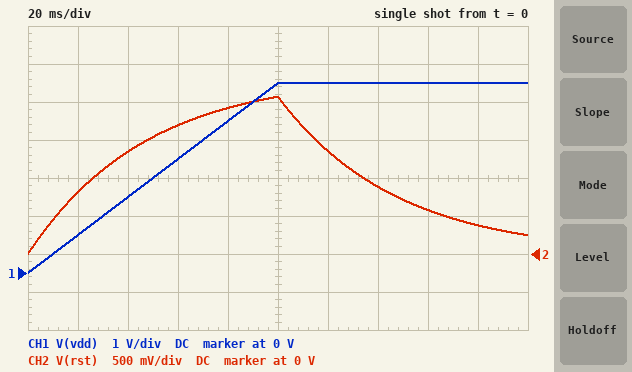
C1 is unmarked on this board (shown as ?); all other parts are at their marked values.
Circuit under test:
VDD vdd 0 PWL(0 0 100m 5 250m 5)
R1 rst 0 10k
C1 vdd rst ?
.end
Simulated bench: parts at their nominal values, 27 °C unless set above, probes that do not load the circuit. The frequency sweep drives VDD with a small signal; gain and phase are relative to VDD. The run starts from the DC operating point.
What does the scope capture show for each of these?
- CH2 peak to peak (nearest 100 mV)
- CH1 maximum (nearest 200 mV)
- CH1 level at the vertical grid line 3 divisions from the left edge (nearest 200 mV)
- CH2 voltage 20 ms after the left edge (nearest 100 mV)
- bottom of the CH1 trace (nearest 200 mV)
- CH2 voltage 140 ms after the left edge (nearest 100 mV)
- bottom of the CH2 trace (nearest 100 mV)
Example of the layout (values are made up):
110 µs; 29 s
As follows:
2.1 V; 5.0 V; 3.0 V; 800 mV; 0 V; 900 mV; 0 V
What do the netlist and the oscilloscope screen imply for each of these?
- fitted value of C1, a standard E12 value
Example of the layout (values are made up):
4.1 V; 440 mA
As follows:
4.7 µF
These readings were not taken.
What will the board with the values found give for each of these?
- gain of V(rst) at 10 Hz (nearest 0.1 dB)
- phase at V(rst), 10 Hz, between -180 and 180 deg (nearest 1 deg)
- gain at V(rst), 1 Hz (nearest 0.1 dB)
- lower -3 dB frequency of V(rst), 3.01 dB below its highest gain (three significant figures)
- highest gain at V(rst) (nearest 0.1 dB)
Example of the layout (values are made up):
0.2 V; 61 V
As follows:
-0.5 dB; 19 deg; -11.0 dB; 3.39 Hz; 0 dB
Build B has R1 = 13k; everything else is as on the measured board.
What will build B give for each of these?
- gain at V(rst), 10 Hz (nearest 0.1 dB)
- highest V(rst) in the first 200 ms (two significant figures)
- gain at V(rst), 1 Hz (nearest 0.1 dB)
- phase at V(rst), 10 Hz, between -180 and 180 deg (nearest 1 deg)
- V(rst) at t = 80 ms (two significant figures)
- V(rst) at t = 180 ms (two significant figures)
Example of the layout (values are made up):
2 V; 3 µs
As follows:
-0.3 dB; 2.5 V; -8.9 dB; 15 deg; 2.2 V; 660 mV
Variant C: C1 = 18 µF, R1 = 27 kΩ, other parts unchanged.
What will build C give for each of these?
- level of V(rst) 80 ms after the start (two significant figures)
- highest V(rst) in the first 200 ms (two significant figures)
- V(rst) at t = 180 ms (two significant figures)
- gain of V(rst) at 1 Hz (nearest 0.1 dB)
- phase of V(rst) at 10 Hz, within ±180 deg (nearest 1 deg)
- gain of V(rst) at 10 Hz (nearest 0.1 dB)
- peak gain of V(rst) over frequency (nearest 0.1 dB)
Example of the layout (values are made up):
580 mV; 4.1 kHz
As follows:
3.7 V; 4.5 V; 3.8 V; -0.4 dB; 2 deg; 0 dB; 0 dB
